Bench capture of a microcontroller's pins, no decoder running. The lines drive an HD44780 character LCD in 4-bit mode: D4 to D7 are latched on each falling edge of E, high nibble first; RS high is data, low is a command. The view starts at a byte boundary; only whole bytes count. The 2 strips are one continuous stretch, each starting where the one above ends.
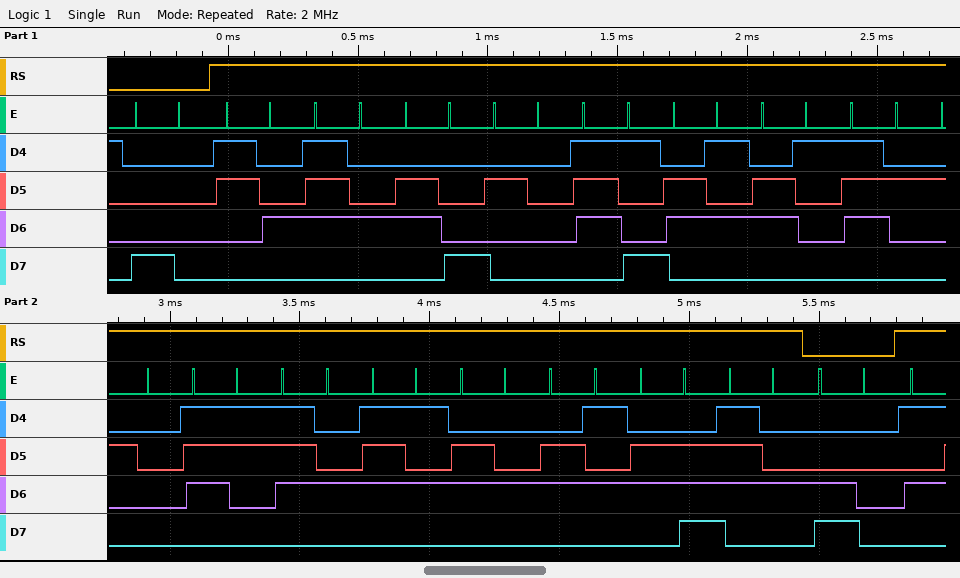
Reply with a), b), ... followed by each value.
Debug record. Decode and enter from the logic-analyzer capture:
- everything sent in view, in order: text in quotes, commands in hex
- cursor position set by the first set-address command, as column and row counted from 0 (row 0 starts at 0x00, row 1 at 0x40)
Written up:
a) 0x80 "4th year student" 0xC0
b) column 0, row 0
